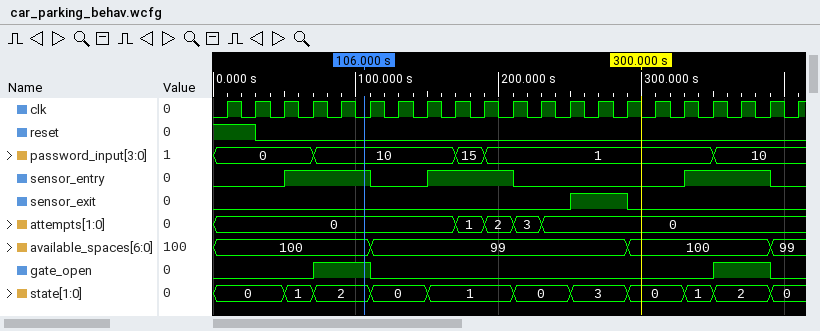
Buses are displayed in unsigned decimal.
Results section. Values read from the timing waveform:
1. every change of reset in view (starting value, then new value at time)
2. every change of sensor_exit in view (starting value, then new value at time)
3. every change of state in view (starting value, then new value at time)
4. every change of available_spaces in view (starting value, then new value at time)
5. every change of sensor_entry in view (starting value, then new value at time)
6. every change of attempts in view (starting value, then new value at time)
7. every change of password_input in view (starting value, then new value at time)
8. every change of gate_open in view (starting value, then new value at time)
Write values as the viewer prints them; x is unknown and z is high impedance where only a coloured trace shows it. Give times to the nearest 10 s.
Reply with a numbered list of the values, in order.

1. 1, 0 at 30 s
2. 0, 1 at 250 s, 0 at 290 s
3. 0, 1 at 50 s, 2 at 70 s, 0 at 110 s, 1 at 150 s, 0 at 210 s, 3 at 250 s, 0 at 290 s, 1 at 330 s, 2 at 350 s, 0 at 390 s
4. 100, 99 at 110 s, 100 at 290 s, 99 at 390 s
5. 0, 1 at 50 s, 0 at 110 s, 1 at 150 s, 0 at 210 s, 1 at 330 s, 0 at 390 s
6. 0, 1 at 170 s, 2 at 190 s, 3 at 210 s, 0 at 230 s
7. 0, 10 at 70 s, 15 at 170 s, 1 at 190 s, 10 at 350 s
8. 0, 1 at 70 s, 0 at 110 s, 1 at 350 s, 0 at 390 s
